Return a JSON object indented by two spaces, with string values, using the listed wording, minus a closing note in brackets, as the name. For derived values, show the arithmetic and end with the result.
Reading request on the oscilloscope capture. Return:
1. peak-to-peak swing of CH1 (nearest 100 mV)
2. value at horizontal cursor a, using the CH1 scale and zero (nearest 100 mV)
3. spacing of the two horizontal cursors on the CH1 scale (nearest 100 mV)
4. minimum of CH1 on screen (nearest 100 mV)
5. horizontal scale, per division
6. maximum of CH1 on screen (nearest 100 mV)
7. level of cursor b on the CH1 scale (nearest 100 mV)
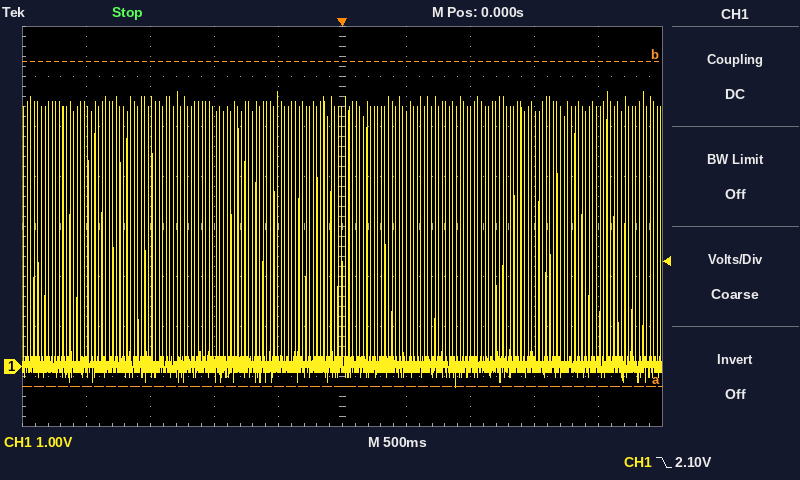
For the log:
{
  "peak-to-peak swing of CH1": "5.5 V − (-400 mV) = 5.9 V",
  "value at horizontal cursor a, using the CH1 scale and zero": "-400 mV",
  "spacing of the two horizontal cursors on the CH1 scale": "6.5 V",
  "minimum of CH1 on screen": "-400 mV",
  "horizontal scale, per division": "500 ms",
  "maximum of CH1 on screen": "5.5 V",
  "level of cursor b on the CH1 scale": "6.1 V"
}
